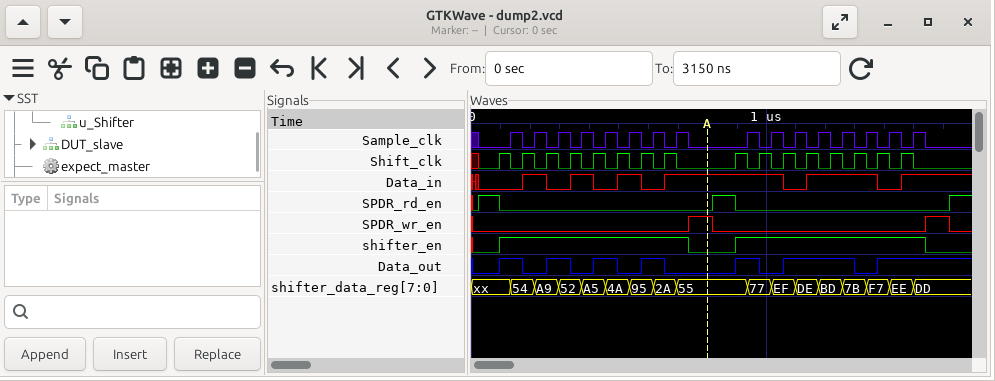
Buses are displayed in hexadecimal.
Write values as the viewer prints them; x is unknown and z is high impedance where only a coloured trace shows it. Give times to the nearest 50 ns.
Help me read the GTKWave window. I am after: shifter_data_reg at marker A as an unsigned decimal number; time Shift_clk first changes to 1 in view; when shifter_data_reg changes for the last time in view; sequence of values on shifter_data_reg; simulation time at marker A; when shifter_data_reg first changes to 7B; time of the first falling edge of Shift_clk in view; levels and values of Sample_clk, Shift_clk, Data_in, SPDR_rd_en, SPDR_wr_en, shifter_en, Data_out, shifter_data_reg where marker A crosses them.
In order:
85
100 ns
1500 ns
xx, 54, A9, 52, A5, 4A, 95, 2A, 55, 77, EF, DE, BD, 7B, F7, EE, DD
800 ns
1250 ns
150 ns
Sample_clk=0, Shift_clk=0, Data_in=1, SPDR_rd_en=0, SPDR_wr_en=1, shifter_en=0, Data_out=0, shifter_data_reg=55
